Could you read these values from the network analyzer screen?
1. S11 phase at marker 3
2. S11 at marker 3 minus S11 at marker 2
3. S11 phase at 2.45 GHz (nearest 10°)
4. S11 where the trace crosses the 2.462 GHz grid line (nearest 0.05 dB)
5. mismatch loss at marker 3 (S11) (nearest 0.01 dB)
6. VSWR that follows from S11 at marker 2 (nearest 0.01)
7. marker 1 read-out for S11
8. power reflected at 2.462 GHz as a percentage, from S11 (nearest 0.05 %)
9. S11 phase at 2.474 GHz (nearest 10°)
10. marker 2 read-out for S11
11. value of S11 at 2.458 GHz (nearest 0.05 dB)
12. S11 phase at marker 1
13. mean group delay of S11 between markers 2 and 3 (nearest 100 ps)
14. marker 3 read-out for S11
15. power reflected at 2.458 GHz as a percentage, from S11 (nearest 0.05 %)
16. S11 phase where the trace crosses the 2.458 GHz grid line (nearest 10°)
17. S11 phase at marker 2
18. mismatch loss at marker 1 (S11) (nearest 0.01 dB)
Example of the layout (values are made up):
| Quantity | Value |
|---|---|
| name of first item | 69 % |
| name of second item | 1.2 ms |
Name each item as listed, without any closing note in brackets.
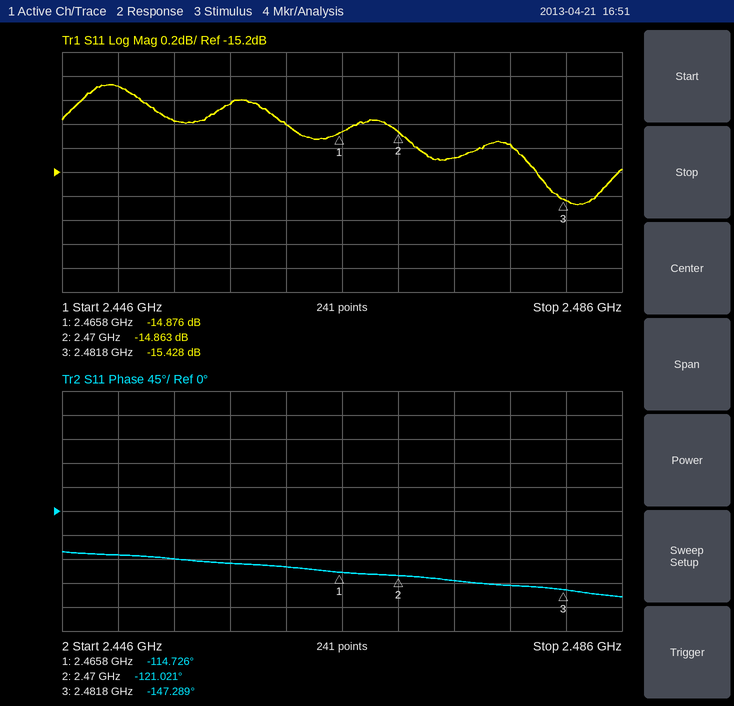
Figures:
| Quantity | Value |
|---|---|
| S11 phase at marker 3 | -147.289° |
| S11 at marker 3 minus S11 at marker 2 | -0.565 dB |
| S11 phase at 2.45 GHz | -80° |
| S11 where the trace crosses the 2.462 GHz grid line | -14.80 dB |
| mismatch loss at marker 3 (S11) | 0.13 dB |
| VSWR that follows from S11 at marker 2 | 1.44 |
| marker 1 read-out for S11 | -14.876 dB |
| power reflected at 2.462 GHz as a percentage, from S11 | 3.30 % |
| S11 phase at 2.474 GHz | -130° |
| marker 2 read-out for S11 | -14.863 dB |
| value of S11 at 2.458 GHz | -14.65 dB |
| S11 phase at marker 1 | -114.726° |
| mean group delay of S11 between markers 2 and 3 | 6.2 ns |
| marker 3 read-out for S11 | -15.428 dB |
| power reflected at 2.458 GHz as a percentage, from S11 | 3.45 % |
| S11 phase where the trace crosses the 2.458 GHz grid line | -100° |
| S11 phase at marker 2 | -121.021° |
| mismatch loss at marker 1 (S11) | 0.14 dB |
